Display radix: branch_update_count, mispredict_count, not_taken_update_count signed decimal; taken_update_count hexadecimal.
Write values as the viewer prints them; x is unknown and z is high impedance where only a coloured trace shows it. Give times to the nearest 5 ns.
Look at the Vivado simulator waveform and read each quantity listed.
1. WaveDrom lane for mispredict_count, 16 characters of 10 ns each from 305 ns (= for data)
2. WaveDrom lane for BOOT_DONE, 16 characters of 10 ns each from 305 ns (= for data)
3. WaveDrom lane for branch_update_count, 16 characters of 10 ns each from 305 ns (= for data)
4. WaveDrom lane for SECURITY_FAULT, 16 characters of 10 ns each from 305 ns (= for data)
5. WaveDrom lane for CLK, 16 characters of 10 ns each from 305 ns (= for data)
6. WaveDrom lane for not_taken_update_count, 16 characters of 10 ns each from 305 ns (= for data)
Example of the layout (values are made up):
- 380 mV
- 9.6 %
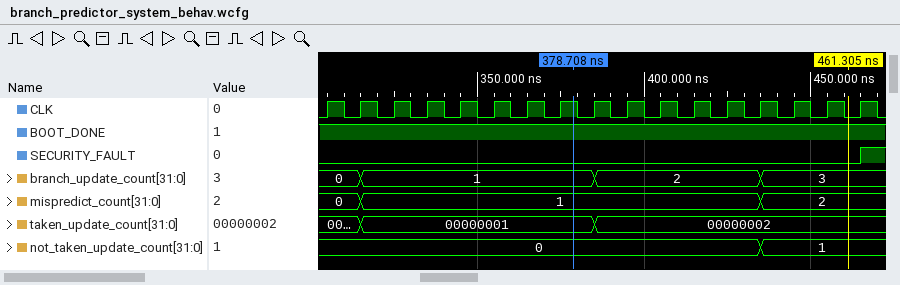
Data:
- {name: 'mispredict_count', wave: '==...........=..', data: '0 1 2'}
- {name: 'BOOT_DONE', wave: '1...............'}
- {name: 'branch_update_count', wave: '==......=....=..', data: '0 1 2 3'}
- {name: 'SECURITY_FAULT', wave: '0...............'}
- {name: 'CLK', wave: 'p...............'}
- {name: 'not_taken_update_count', wave: '=............=..', data: '0 1'}
